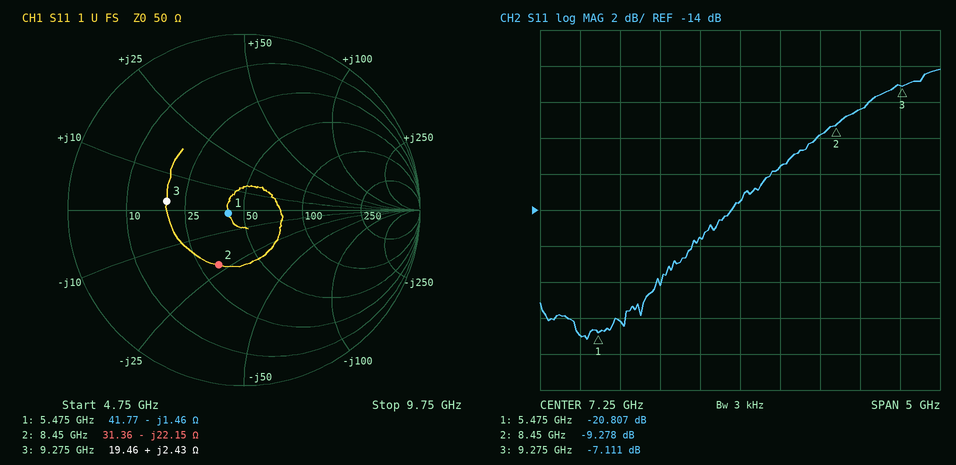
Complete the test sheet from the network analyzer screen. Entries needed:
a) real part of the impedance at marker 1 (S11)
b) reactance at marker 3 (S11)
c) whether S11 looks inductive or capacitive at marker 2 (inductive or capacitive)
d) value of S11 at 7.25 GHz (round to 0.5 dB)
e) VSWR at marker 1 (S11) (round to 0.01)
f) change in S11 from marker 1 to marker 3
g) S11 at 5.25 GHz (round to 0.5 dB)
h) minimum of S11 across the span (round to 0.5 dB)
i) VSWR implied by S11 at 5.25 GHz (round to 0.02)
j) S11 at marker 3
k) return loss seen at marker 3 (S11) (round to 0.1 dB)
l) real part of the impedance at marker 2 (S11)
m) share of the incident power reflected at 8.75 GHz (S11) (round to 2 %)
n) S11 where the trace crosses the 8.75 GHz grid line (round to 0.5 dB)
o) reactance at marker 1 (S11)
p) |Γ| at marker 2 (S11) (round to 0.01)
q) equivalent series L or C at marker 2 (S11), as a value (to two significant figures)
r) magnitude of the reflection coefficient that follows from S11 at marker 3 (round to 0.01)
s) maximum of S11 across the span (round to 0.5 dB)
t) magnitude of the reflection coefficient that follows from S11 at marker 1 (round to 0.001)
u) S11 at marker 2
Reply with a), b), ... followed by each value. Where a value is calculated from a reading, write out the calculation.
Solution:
a) 41.77 Ω
b) +2.43 Ω
c) capacitive
d) -13.5 dB
e) 1.20
f) -7.111 − (-20.807) = 13.696 dB
g) -21.0 dB
h) -21.0 dB
i) |Γ| = 10^(-21/20) = 0.0891; VSWR = (1 + 0.0891)/(1 − 0.0891) ≈ 1.20
j) -7.111 dB
k) 7.1 dB
l) 31.36 Ω
m) 10^(-8.5/10) ≈ 14 %
n) -8.5 dB
o) -1.46 Ω
p) 0.34
q) C = 1/(2π × 8.45 GHz × 22.15 Ω) ≈ 850 fF
r) 10^(-7.111/20) ≈ 0.44
s) -6.0 dB
t) 10^(-20.807/20) ≈ 0.091
u) -9.278 dB
